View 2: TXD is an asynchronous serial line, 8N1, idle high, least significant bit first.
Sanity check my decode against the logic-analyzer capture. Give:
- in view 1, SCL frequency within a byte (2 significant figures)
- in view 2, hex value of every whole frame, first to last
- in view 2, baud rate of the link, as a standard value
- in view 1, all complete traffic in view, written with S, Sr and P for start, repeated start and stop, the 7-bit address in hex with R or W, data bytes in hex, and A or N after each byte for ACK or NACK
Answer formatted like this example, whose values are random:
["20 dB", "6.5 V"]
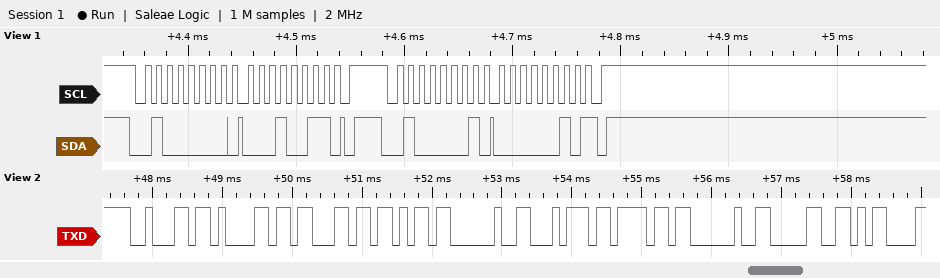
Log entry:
["100 kHz", "62 61 63 6B 20 74 6F 20 30 0D", "9600 baud", "S 20W A 13 A P S 20R A 02 N P"]
